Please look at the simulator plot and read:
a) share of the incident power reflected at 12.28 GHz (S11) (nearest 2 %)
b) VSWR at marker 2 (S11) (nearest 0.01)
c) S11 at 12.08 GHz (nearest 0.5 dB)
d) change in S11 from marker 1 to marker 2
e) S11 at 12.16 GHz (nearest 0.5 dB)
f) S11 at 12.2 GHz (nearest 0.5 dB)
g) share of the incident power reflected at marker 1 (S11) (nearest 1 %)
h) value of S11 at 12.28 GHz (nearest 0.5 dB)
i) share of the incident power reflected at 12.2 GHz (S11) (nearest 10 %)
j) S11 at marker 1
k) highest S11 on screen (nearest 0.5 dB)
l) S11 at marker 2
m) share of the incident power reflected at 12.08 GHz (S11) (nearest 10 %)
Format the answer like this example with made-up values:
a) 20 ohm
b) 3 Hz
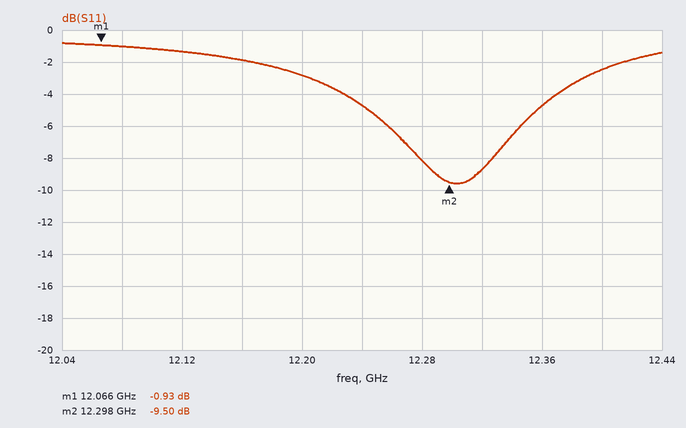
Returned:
a) 16 %
b) 2.01
c) -1.0 dB
d) -8.57 dB
e) -2.0 dB
f) -3.0 dB
g) 81 %
h) -8.0 dB
i) 50 %
j) -0.93 dB
k) -1.0 dB
l) -9.50 dB
m) 80 %
